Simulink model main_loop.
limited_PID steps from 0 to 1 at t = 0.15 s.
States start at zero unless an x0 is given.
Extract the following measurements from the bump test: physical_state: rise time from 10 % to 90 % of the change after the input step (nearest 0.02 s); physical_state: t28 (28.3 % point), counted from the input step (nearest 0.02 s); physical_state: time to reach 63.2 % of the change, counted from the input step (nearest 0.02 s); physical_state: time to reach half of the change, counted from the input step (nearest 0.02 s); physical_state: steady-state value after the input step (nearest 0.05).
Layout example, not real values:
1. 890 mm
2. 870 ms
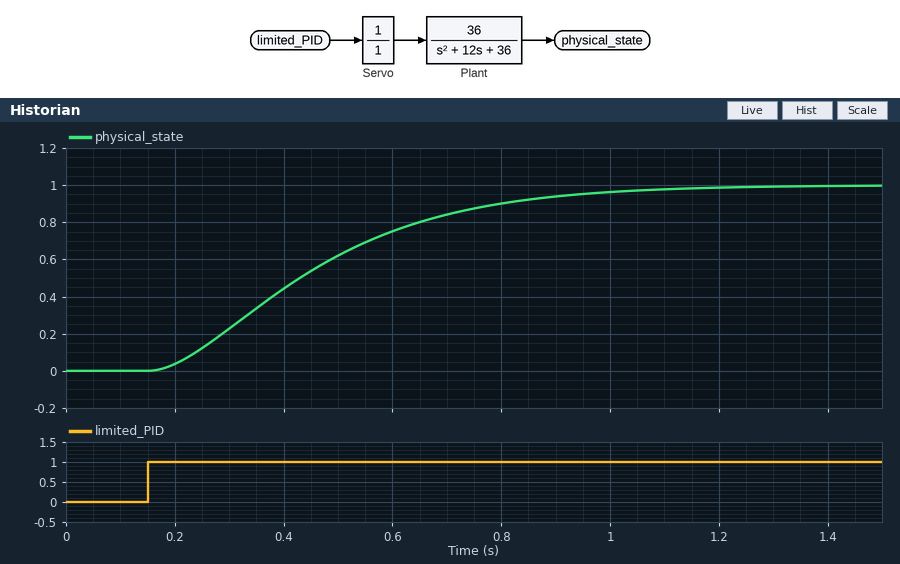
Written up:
1. 0.56 s
2. 0.18 s
3. 0.36 s
4. 0.28 s
5. 1.00
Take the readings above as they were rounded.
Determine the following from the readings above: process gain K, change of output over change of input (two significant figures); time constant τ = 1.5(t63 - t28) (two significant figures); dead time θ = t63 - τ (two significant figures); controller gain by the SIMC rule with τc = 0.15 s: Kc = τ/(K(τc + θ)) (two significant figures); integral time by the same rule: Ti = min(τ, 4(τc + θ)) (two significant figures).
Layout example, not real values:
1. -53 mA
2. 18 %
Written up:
1. 1.0
2. 0.27 s
3. 0.090 s
4. 1.1
5. 0.27 s
